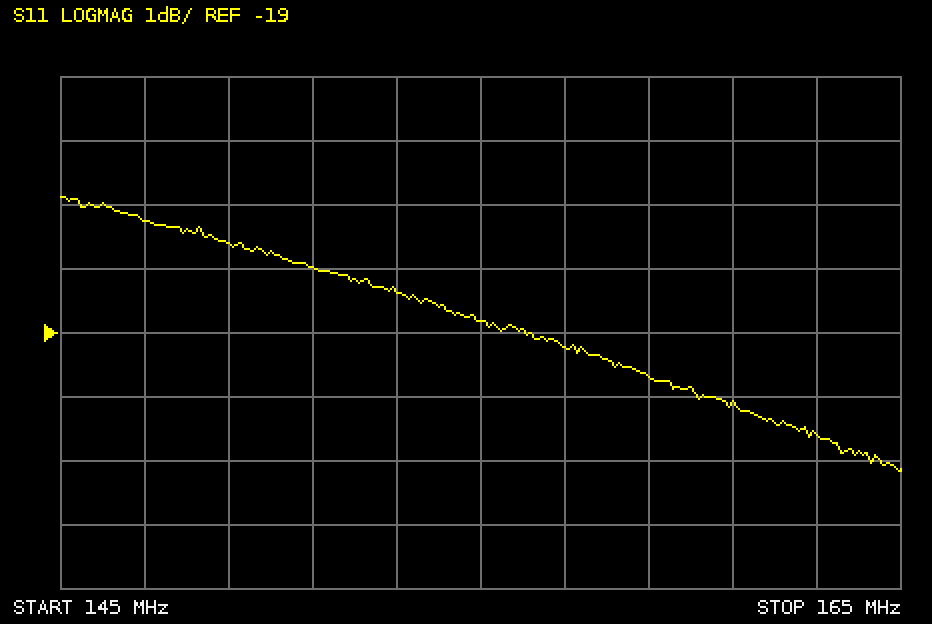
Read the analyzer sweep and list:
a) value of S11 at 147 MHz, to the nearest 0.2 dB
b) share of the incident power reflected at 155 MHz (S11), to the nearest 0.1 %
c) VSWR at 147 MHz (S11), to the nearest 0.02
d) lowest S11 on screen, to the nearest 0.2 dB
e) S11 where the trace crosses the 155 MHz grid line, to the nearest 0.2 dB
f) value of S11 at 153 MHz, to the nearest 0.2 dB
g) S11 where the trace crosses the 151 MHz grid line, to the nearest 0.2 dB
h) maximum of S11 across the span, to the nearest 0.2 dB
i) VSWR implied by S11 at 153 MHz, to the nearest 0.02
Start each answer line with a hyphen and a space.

- -17.2 dB
- 1.3 %
- 1.32
- -21.2 dB
- -18.8 dB
- -18.4 dB
- -18.0 dB
- -16.8 dB
- 1.28
